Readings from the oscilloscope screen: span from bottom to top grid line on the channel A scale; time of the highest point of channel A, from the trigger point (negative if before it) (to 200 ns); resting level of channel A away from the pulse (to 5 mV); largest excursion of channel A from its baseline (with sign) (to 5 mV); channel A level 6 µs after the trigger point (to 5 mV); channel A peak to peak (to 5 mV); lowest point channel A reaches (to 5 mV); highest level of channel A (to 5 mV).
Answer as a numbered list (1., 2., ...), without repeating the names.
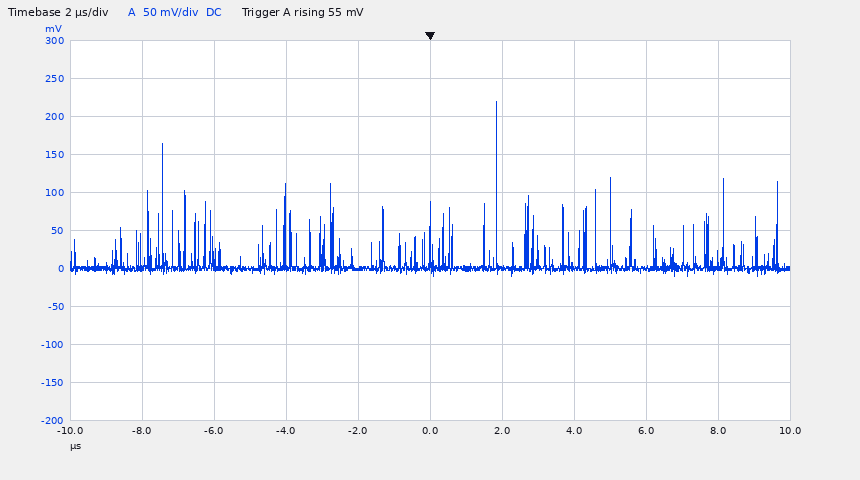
1. 500 mV
2. +1.8 µs
3. 0 mV
4. +220 mV
5. 0 mV
6. 230 mV
7. -10 mV
8. 220 mV
